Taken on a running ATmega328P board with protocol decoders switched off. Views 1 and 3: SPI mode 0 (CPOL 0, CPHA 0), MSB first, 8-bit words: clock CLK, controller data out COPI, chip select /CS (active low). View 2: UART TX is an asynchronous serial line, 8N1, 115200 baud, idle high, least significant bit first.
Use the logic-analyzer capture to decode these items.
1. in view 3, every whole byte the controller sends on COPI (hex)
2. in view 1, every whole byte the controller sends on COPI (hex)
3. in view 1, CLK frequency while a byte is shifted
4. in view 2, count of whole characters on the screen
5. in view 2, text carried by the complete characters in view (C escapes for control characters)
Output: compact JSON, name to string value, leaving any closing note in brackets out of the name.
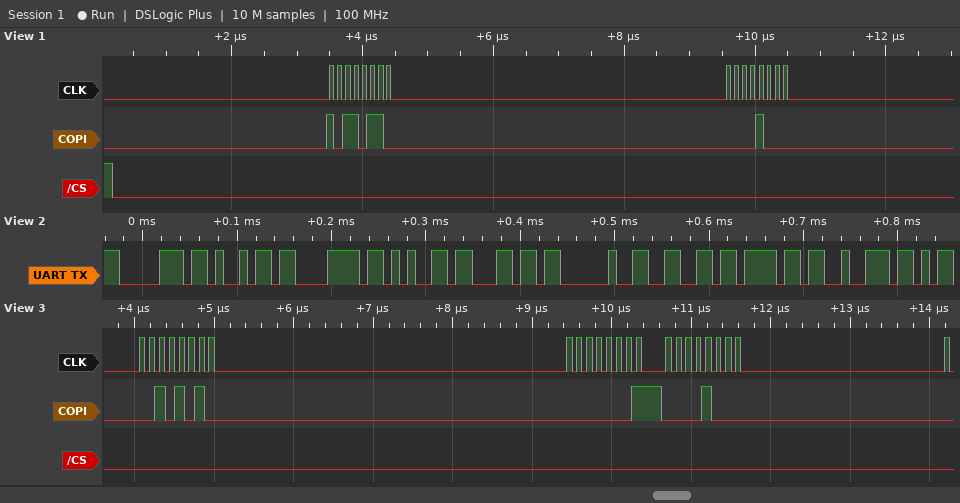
{"in view 3, every whole byte the controller sends on COPI": "2A 01 08", "in view 1, every whole byte the controller sends on COPI": "0xB6 0x08", "in view 1, CLK frequency while a byte is shifted": "8 MHz", "in view 2, count of whole characters on the screen": "9", "in view 2, text carried by the complete characters in view": "\"pixel for\""}
